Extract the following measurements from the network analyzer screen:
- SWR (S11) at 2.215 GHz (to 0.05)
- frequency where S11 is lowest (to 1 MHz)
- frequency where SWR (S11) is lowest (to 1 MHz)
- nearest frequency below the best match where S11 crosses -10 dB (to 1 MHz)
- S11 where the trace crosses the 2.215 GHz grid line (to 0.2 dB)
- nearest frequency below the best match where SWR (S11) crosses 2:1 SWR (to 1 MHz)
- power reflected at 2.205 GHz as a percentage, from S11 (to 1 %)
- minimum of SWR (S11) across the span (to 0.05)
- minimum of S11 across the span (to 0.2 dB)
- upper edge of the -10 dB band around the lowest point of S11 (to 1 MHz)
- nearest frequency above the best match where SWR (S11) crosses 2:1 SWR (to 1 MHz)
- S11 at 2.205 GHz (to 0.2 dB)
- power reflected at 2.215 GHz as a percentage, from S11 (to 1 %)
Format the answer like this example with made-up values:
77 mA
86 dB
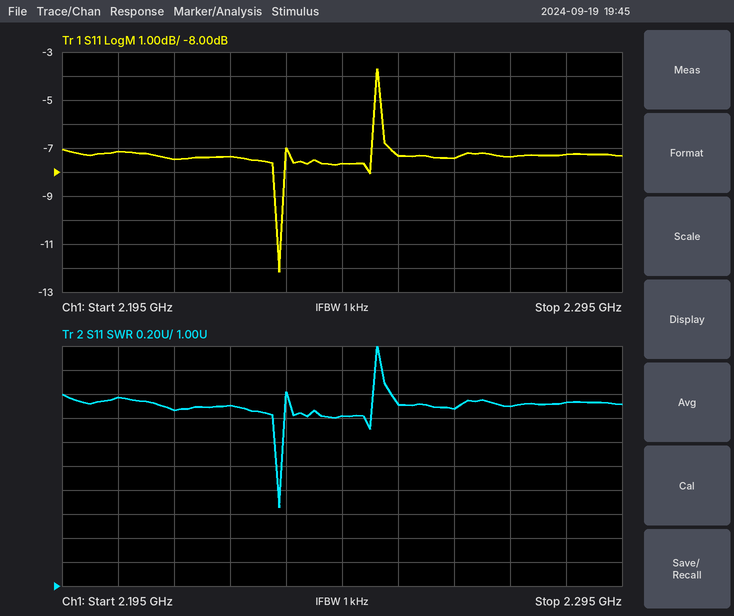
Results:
2.45
2.234 GHz
2.234 GHz
2.233 GHz
-7.4 dB
2.233 GHz
19 %
1.65
-12.2 dB
2.234 GHz
2.234 GHz
-7.2 dB
18 %
